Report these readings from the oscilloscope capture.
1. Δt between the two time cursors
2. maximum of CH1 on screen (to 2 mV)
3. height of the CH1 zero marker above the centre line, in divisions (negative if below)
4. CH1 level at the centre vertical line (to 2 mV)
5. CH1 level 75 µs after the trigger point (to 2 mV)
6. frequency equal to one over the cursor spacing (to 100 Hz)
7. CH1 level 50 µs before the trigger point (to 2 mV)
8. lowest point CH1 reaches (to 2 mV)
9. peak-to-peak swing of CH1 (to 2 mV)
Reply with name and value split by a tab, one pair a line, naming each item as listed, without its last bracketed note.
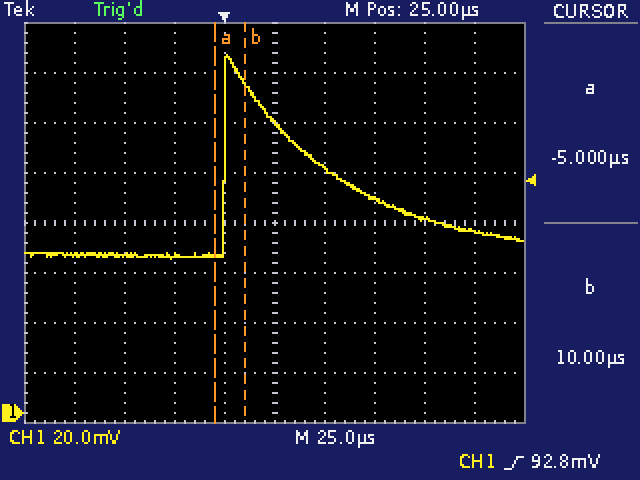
Δt between the two time cursors	15.0 µs
maximum of CH1 on screen	144 mV
height of the CH1 zero marker above the centre line, in divisions	-3.8 div
CH1 level at the centre vertical line	116 mV
CH1 level 75 µs after the trigger point	86 mV
frequency equal to one over the cursor spacing	66.7 kHz
CH1 level 50 µs before the trigger point	64 mV
lowest point CH1 reaches	62 mV
peak-to-peak swing of CH1	82 mV
